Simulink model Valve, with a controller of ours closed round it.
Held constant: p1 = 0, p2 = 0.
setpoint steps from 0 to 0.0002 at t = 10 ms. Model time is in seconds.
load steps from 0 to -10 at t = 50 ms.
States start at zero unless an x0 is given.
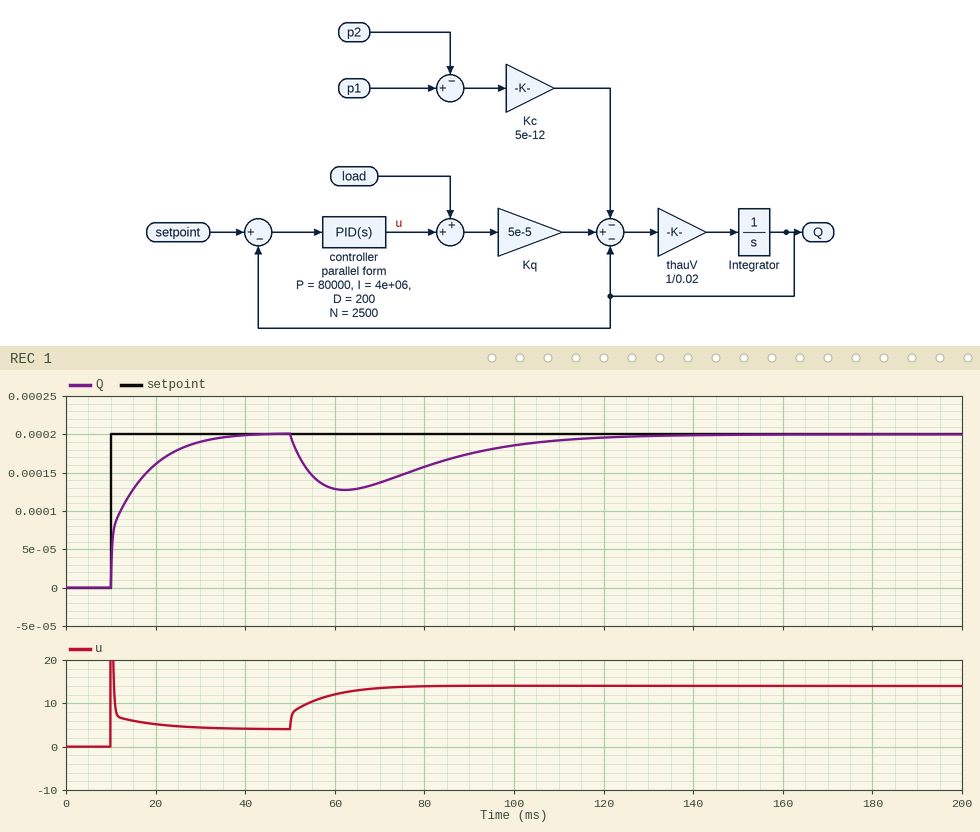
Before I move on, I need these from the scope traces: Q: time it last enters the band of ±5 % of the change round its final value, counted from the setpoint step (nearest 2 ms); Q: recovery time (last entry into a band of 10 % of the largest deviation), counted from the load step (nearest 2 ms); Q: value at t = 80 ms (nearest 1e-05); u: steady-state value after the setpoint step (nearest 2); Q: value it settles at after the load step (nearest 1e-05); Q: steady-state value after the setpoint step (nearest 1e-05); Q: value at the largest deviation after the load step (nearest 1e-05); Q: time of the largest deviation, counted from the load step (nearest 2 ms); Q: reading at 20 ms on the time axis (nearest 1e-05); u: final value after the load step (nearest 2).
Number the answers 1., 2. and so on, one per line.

1. 20 ms
2. 62 ms
3. 0.00016
4. 4
5. 0.00020
6. 0.00020
7. 0.00013
8. 12 ms
9. 0.00016
10. 14
